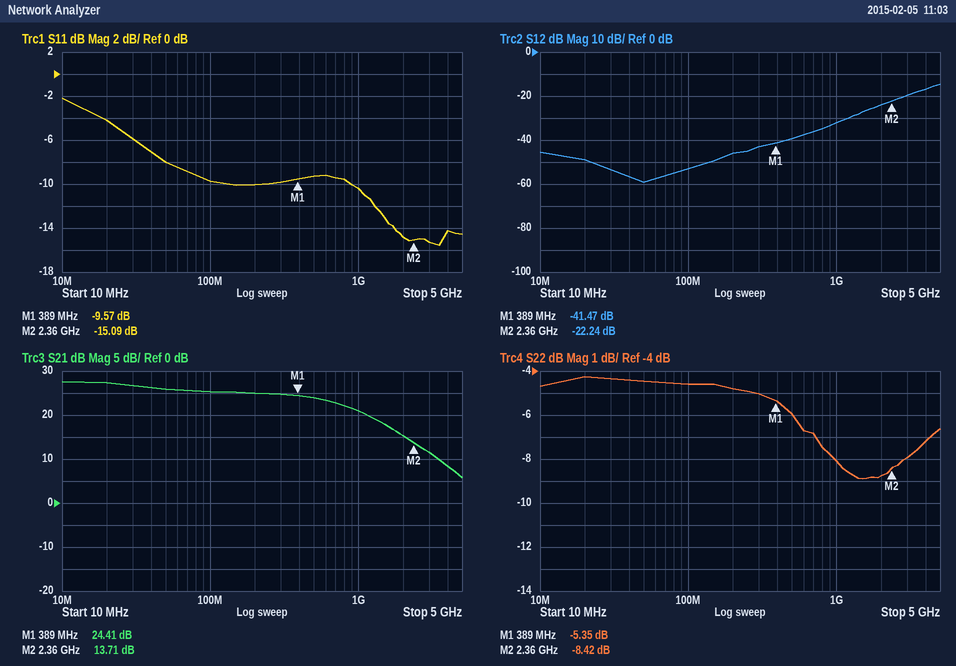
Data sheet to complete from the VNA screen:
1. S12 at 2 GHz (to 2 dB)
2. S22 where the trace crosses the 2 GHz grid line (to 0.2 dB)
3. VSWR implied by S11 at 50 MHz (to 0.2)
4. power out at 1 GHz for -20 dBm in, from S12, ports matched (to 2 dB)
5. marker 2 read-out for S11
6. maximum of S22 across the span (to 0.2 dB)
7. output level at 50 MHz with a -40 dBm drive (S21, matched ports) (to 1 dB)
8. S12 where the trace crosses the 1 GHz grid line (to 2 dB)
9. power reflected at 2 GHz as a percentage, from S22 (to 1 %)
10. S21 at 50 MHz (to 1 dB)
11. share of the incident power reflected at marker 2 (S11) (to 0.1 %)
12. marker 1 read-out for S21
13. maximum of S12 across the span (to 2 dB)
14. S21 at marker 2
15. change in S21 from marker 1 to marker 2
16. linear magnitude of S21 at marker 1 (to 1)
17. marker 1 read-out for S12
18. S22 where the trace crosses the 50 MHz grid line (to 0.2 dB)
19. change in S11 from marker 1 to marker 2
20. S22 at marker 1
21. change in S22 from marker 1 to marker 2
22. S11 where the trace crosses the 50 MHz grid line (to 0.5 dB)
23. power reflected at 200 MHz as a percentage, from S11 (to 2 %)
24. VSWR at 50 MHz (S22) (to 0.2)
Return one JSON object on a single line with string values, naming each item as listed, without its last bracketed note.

{"S12 at 2 GHz": "-24 dB", "S22 where the trace crosses the 2 GHz grid line": "-8.8 dB", "VSWR implied by S11 at 50 MHz": "2.4", "power out at 1 GHz for -20 dBm in, from S12, ports matched": "-52 dBm", "marker 2 read-out for S11": "-15.09 dB", "maximum of S22 across the span": "-4.2 dB", "output level at 50 MHz with a -40 dBm drive (S21, matched ports)": "-14 dBm", "S12 where the trace crosses the 1 GHz grid line": "-32 dB", "power reflected at 2 GHz as a percentage, from S22": "13 %", "S21 at 50 MHz": "26 dB", "share of the incident power reflected at marker 2 (S11)": "3.1 %", "marker 1 read-out for S21": "24.41 dB", "maximum of S12 across the span": "-14 dB", "S21 at marker 2": "13.71 dB", "change in S21 from marker 1 to marker 2": "-10.70 dB", "linear magnitude of S21 at marker 1": "17", "marker 1 read-out for S12": "-41.47 dB", "S22 where the trace crosses the 50 MHz grid line": "-4.4 dB", "change in S11 from marker 1 to marker 2": "-5.52 dB", "S22 at marker 1": "-5.35 dB", "change in S22 from marker 1 to marker 2": "-3.07 dB", "S11 where the trace crosses the 50 MHz grid line": "-8.0 dB", "power reflected at 200 MHz as a percentage, from S11": "10 %", "VSWR at 50 MHz (S22)": "4.0"}
